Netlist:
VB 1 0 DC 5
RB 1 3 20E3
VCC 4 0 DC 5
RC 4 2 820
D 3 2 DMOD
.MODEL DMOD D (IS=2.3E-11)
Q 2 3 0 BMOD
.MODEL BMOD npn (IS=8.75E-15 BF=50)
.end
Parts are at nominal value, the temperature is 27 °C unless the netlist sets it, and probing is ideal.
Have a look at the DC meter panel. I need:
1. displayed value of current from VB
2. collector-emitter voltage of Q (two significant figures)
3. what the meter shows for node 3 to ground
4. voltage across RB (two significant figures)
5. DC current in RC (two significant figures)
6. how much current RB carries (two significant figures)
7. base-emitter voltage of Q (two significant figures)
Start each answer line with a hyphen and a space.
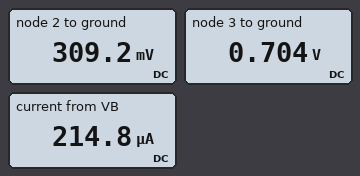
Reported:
- 214.8 µA
- 310 mV
- 0.704 V
- 4.3 V
- 5.7 mA
- 210 µA
- 700 mV
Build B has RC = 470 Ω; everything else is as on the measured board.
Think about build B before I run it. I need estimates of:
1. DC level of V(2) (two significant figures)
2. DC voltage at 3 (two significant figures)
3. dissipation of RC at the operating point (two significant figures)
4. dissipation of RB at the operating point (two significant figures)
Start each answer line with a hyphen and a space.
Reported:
- 370 mV
- 720 mV
- 46 mW
- 920 µW
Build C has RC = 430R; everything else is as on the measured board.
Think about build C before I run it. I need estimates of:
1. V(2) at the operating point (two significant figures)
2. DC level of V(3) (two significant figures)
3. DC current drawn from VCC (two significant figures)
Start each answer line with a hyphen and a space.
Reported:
- 430 mV
- 720 mV
- 11 mA
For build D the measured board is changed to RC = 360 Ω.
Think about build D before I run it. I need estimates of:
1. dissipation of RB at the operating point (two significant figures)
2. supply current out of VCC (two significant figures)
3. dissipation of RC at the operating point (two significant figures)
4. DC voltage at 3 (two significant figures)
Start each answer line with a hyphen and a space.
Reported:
- 920 µW
- 11 mA
- 41 mW
- 720 mV
